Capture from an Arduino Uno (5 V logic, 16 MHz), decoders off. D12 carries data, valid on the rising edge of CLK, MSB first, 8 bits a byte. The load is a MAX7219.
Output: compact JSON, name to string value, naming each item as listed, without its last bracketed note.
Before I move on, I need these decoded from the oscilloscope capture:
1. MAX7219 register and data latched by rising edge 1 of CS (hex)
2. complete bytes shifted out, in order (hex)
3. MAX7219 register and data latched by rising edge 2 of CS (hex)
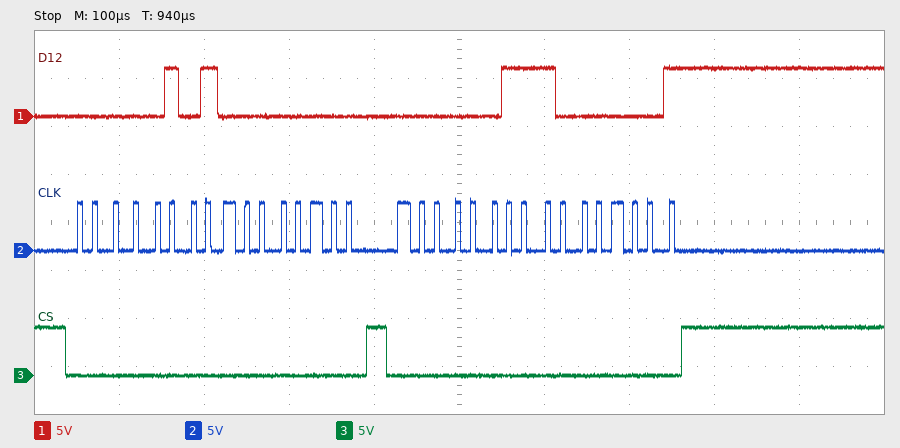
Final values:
{"MAX7219 register and data latched by rising edge 1 of CS": "register 0x5, data 0x00", "complete bytes shifted out, in order": "05 00 03 81", "MAX7219 register and data latched by rising edge 2 of CS": "register 0x3, data 0x81"}
